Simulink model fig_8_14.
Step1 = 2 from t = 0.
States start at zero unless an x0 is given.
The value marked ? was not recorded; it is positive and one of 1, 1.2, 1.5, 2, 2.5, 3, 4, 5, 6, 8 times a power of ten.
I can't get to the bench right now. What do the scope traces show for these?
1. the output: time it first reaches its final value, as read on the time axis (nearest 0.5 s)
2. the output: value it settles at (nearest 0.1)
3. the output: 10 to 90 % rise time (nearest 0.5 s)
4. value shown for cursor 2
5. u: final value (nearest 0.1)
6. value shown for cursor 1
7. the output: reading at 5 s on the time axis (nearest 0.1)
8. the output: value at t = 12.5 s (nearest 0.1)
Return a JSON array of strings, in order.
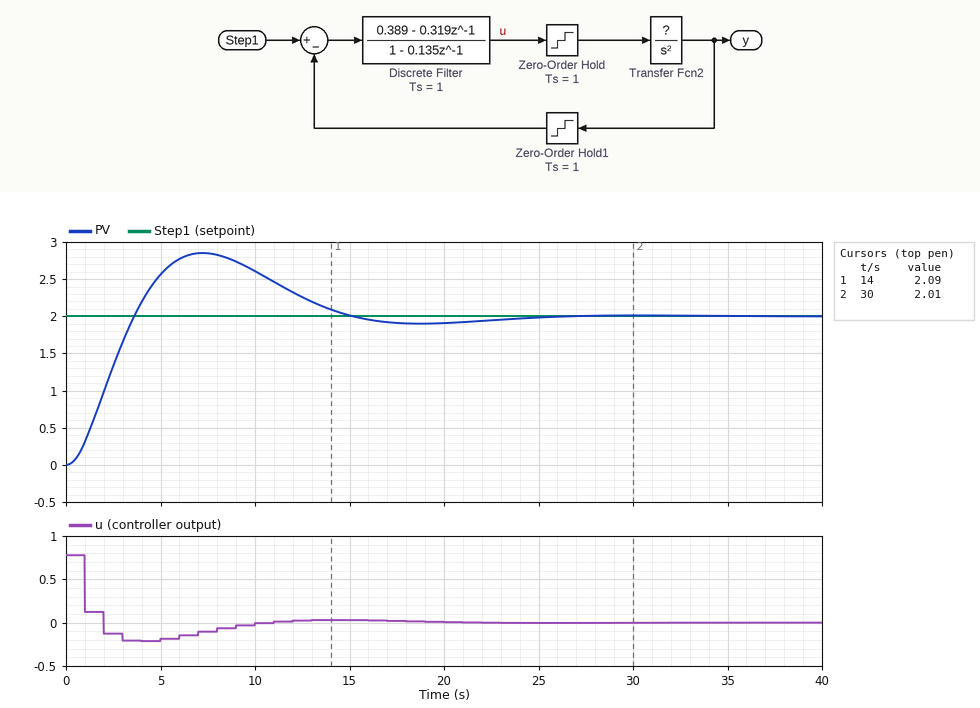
["3.5 s", "2.0", "2.5 s", "2.01", "0.0", "2.09", "2.6", "2.3"]
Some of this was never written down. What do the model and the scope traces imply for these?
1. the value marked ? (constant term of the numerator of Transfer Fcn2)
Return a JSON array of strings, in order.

["0.8"]
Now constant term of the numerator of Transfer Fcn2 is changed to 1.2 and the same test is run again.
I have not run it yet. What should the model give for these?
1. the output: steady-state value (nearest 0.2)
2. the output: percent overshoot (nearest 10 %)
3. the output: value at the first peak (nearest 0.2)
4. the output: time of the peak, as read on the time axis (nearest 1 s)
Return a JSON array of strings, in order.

["2.0", "50 %", "3.0", "5 s"]
